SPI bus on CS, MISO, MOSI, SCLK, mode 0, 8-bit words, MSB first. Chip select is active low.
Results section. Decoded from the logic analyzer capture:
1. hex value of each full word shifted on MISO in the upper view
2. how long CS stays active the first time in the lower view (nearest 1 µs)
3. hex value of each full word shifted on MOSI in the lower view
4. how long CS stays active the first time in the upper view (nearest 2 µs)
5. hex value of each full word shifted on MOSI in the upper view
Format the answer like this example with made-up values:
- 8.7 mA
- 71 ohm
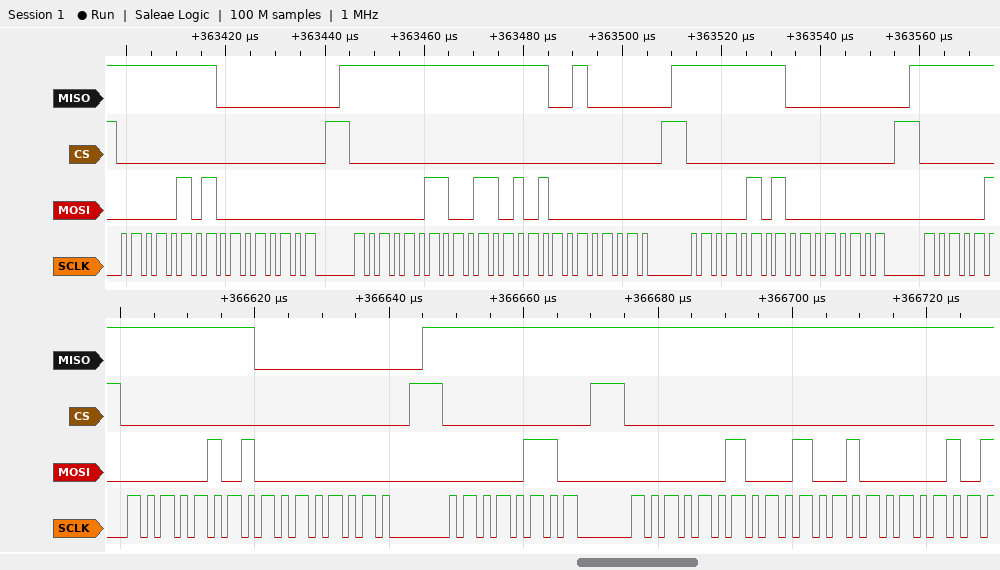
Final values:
- FF, 00, FF, FF, 20, FF, 00
- 43 µs
- 05, 00, 06, 02, 24
- 42 µs
- 05, 00, 03, 35, 00, 05, 00
